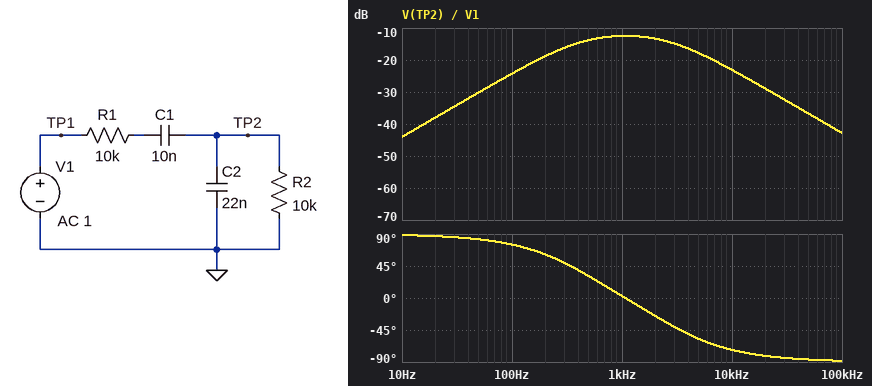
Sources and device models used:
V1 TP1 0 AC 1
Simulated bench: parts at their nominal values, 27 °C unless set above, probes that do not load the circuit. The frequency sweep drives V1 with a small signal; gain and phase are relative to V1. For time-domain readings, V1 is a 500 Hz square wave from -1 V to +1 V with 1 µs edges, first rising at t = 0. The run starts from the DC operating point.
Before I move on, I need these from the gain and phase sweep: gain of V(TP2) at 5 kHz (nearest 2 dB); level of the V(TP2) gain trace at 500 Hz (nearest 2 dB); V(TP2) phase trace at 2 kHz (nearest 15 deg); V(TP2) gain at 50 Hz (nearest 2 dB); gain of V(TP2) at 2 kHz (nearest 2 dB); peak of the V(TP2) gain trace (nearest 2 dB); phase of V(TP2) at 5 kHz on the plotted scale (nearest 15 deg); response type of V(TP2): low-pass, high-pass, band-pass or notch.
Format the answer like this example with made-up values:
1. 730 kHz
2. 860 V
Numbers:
1. -18 dB
2. -14 dB
3. -30 deg
4. -30 dB
5. -14 dB
6. -12 dB
7. -60 deg
8. band-pass
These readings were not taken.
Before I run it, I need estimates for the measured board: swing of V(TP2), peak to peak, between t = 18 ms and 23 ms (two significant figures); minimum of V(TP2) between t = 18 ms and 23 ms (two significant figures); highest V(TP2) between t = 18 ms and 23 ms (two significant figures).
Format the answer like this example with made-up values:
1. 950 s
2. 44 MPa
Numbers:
1. 720 mV
2. -360 mV
3. 360 mV
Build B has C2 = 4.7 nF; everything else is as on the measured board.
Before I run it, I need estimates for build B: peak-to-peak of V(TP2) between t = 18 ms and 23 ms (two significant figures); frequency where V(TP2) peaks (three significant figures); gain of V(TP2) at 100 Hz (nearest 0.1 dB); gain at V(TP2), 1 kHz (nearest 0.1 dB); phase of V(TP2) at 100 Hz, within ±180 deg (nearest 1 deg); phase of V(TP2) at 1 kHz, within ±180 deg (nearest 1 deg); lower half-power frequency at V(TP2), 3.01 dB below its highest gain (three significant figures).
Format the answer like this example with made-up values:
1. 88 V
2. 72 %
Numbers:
1. 1.4 V
2. 2.32 kHz
3. -24.1 dB
4. -8.9 dB
5. 81 deg
6. 28 deg
7. 601 Hz
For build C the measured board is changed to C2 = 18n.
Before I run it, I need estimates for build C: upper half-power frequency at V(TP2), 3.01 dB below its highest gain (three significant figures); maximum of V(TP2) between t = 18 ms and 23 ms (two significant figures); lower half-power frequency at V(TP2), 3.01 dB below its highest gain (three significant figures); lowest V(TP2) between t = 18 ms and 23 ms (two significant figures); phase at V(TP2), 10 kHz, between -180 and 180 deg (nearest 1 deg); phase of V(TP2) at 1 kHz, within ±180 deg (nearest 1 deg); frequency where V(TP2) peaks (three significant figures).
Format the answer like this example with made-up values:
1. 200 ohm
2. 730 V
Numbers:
1. 3.74 kHz
2. 410 mV
3. 377 Hz
4. -410 mV
5. -71 deg
6. 7 deg
7. 1.19 kHz
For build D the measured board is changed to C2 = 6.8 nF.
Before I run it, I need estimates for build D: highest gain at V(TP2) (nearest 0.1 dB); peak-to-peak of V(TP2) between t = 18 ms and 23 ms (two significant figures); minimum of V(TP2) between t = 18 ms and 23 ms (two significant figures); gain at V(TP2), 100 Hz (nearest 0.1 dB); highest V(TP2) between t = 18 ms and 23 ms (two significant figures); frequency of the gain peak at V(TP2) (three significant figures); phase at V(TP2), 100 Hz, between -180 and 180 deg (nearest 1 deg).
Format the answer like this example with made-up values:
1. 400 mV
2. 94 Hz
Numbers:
1. -8.6 dB
2. 1.2 V
3. -620 mV
4. -24.1 dB
5. 620 mV
6. 1.93 kHz
7. 80 deg
